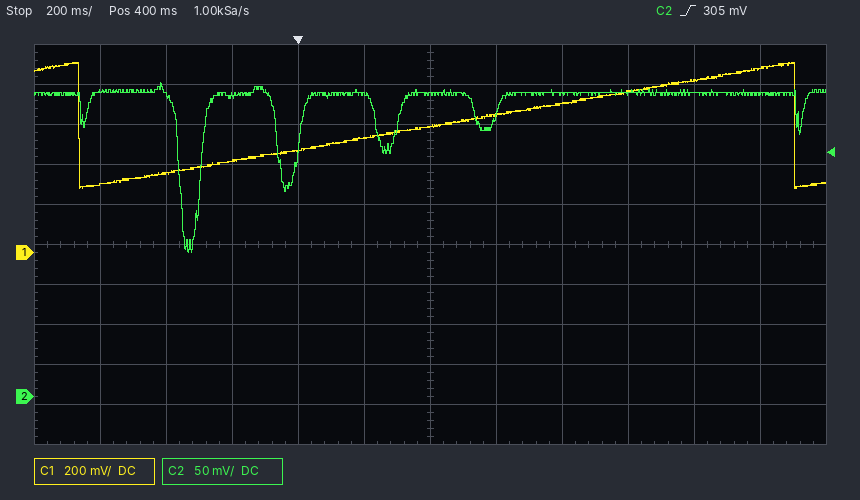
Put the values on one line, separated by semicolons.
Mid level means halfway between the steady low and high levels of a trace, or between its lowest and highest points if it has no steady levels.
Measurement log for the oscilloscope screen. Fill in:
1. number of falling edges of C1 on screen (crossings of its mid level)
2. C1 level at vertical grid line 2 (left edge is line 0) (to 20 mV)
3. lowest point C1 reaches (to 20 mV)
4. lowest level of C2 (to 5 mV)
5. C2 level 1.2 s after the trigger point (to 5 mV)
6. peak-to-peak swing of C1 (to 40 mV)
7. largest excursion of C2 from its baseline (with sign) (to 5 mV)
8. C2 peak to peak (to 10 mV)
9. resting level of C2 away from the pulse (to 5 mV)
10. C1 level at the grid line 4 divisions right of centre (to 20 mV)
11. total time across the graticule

2; 400 mV; 320 mV; 180 mV; 380 mV; 640 mV; -200 mV; 210 mV; 380 mV; 860 mV; 2.4 s
